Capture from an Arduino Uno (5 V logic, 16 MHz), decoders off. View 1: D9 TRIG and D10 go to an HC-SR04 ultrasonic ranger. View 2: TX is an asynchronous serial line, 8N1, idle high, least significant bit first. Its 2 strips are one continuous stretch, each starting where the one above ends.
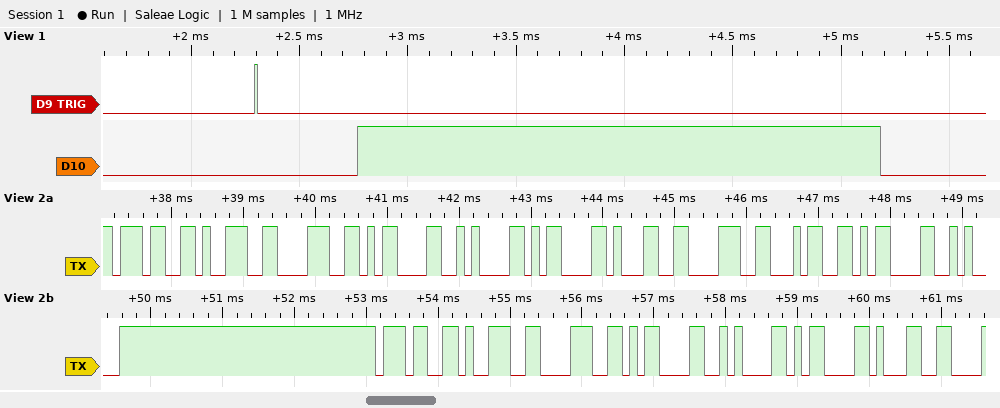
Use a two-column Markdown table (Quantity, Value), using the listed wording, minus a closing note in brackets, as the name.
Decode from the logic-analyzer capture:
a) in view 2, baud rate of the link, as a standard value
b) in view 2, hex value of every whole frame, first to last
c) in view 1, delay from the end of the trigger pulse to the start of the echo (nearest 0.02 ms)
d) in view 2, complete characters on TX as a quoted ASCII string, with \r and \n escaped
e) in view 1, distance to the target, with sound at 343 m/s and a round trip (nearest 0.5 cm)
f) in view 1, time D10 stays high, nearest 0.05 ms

| Quantity | Value |
|---|---|
| in view 2, baud rate of the link, as a standard value | 9600 baud |
| in view 2, hex value of every whole frame, first to last | 37 39 38 0D 0A 0D 31 38 34 0D 0A 37 39 38 0D 0A 0D 31 |
| in view 1, delay from the end of the trigger pulse to the start of the echo | 0.46 ms |
| in view 2, complete characters on TX as a quoted ASCII string, with \r and \n escaped | "798\r\n\r184\r\n798\r\n\r1" |
| in view 1, distance to the target, with sound at 343 m/s and a round trip | 41.5 cm |
| in view 1, time D10 stays high, nearest 0.05 ms | 2.40 ms |
